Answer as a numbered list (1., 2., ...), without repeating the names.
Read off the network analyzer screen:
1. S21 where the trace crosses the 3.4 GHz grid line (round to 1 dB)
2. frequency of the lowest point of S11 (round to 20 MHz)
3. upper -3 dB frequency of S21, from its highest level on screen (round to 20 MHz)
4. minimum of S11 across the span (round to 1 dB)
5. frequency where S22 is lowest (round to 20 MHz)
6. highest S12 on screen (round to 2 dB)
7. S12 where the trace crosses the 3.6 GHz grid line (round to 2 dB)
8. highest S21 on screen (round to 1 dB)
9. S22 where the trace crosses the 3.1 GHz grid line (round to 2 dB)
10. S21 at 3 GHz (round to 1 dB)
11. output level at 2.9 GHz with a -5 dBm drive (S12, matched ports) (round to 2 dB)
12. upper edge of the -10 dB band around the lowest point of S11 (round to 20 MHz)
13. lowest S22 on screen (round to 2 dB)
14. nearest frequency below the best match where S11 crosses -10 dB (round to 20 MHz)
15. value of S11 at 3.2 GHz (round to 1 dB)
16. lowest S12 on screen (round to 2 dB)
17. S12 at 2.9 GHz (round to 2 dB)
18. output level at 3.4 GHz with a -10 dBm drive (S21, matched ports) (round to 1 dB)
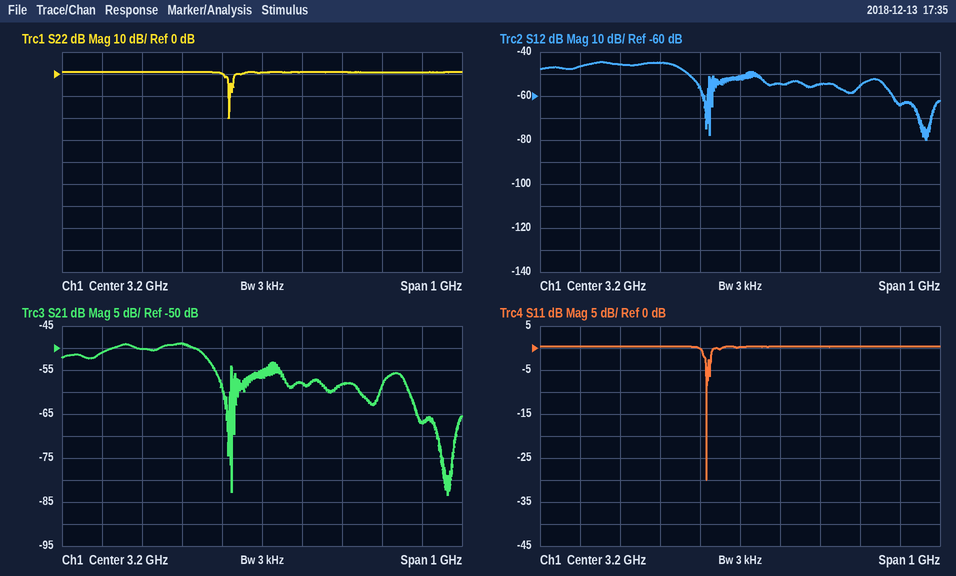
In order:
1. -58 dB
2. 3.12 GHz
3. 3.06 GHz
4. -30 dB
5. 3.12 GHz
6. -44 dB
7. -64 dB
8. -49 dB
9. 0 dB
10. -49 dB
11. -50 dBm
12. 3.12 GHz
13. -20 dB
14. 3.12 GHz
15. 0 dB
16. -80 dB
17. -46 dB
18. -68 dBm
